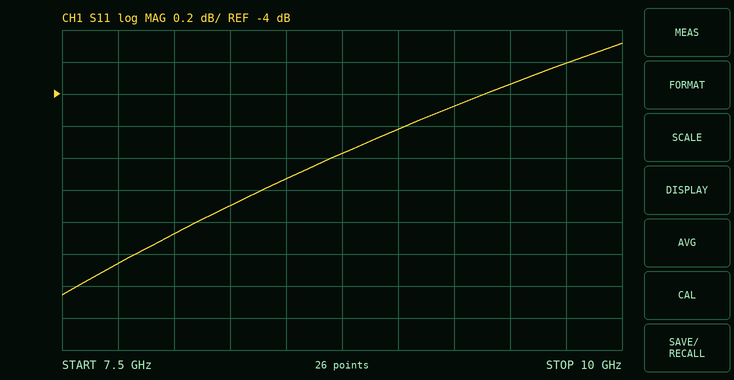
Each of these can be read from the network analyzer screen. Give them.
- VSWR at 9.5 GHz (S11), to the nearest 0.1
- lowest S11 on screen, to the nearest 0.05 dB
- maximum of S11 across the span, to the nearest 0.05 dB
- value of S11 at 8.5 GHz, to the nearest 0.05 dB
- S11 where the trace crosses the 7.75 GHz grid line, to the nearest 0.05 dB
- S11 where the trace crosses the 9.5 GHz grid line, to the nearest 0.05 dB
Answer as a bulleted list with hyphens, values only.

- 4.5
- -5.25 dB
- -3.70 dB
- -4.55 dB
- -5.05 dB
- -3.95 dB
